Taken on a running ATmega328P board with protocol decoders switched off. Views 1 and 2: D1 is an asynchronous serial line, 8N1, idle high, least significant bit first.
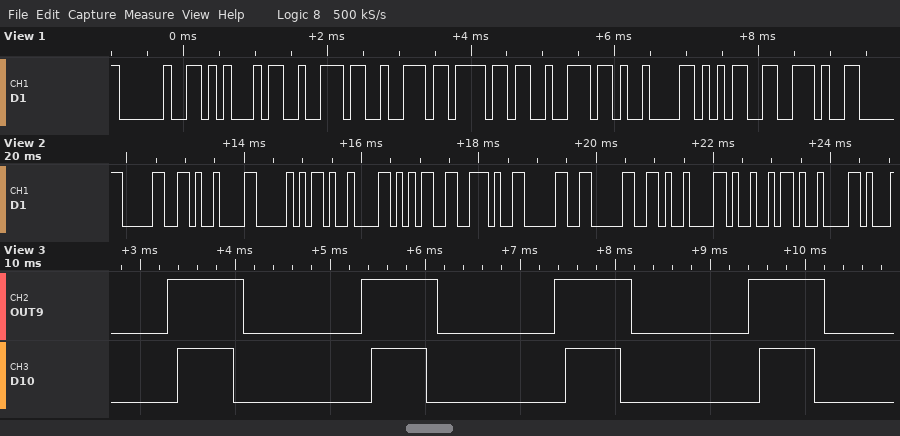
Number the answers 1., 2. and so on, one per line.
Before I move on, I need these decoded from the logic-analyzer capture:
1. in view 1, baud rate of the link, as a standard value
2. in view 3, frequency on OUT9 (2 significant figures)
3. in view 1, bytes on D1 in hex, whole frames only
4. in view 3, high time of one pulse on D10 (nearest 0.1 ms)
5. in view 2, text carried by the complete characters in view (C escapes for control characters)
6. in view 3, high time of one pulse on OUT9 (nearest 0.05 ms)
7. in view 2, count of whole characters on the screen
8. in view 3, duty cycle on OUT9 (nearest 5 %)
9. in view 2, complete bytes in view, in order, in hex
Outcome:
1. 9600 baud
2. 490 Hz
3. 20 45 72 72 6F 72 09 35 2E
4. 0.6 ms
5. "0\tP\t5.00\tI\t"
6. 0.80 ms
7. 11
8. 40 %
9. 30 09 50 09 35 2E 30 30 09 49 09
